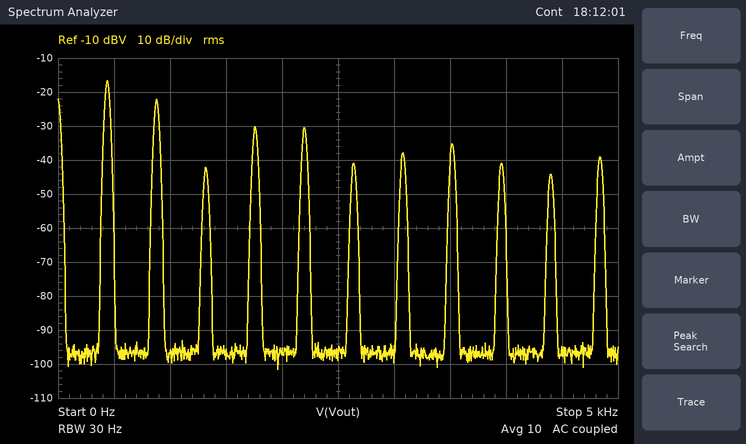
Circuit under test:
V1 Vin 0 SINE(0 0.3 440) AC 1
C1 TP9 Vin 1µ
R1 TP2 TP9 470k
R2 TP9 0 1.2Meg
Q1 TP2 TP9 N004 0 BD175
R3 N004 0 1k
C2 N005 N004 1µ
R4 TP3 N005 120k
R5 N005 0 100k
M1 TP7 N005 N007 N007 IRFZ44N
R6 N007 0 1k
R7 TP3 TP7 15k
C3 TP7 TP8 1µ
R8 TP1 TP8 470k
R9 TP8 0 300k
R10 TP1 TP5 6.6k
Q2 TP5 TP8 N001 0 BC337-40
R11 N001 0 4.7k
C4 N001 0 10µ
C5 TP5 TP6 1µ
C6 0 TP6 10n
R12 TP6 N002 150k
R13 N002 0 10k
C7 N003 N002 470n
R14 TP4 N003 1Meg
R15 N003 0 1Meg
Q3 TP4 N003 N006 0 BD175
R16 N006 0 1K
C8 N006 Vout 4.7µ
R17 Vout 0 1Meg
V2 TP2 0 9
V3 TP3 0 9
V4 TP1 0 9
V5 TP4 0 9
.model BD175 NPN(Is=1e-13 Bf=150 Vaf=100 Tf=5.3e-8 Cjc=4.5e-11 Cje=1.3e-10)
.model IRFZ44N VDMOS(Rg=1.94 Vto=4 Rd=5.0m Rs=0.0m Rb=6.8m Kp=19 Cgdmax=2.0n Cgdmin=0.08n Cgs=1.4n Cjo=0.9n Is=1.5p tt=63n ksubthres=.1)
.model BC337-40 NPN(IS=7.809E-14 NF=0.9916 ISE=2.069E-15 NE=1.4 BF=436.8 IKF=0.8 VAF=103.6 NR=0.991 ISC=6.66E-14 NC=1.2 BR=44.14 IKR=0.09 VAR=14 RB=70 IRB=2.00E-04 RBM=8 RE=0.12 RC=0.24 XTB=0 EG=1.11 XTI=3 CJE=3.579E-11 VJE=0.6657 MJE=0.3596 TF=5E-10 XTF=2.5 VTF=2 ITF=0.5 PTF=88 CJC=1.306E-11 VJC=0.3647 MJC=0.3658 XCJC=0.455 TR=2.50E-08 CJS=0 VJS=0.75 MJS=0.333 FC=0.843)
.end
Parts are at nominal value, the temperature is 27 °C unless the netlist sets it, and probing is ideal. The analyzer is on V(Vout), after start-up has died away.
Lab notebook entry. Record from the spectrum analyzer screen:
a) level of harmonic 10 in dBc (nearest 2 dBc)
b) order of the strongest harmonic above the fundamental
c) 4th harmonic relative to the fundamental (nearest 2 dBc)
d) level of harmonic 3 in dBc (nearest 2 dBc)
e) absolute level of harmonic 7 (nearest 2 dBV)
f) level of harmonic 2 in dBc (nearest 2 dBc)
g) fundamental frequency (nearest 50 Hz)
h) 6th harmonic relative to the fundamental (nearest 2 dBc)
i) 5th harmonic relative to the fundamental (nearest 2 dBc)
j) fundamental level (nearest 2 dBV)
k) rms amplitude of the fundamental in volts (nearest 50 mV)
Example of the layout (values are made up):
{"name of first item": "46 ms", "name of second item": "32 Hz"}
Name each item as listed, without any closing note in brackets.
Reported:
{"level of harmonic 10 in dBc": "-28 dBc", "order of the strongest harmonic above the fundamental": "2", "4th harmonic relative to the fundamental": "-14 dBc", "level of harmonic 3 in dBc": "-26 dBc", "absolute level of harmonic 7": "-38 dBV", "level of harmonic 2 in dBc": "-6 dBc", "fundamental frequency": "450 Hz", "6th harmonic relative to the fundamental": "-24 dBc", "5th harmonic relative to the fundamental": "-14 dBc", "fundamental level": "-16 dBV", "rms amplitude of the fundamental in volts": "150 mV"}
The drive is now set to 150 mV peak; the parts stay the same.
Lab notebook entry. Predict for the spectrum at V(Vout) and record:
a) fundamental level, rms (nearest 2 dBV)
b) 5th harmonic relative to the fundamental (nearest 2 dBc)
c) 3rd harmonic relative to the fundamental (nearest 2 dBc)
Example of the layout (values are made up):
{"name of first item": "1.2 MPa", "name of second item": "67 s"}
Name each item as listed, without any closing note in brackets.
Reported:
{"fundamental level, rms": "-16 dBV", "5th harmonic relative to the fundamental": "-16 dBc", "3rd harmonic relative to the fundamental": "-32 dBc"}
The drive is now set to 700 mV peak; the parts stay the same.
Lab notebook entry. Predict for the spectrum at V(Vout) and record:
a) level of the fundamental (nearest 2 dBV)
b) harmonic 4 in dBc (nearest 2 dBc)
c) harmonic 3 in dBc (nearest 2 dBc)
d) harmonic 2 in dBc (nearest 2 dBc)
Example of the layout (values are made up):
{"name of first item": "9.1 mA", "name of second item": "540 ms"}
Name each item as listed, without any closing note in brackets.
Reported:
{"level of the fundamental": "-16 dBV", "harmonic 4 in dBc": "-12 dBc", "harmonic 3 in dBc": "-24 dBc", "harmonic 2 in dBc": "-8 dBc"}
